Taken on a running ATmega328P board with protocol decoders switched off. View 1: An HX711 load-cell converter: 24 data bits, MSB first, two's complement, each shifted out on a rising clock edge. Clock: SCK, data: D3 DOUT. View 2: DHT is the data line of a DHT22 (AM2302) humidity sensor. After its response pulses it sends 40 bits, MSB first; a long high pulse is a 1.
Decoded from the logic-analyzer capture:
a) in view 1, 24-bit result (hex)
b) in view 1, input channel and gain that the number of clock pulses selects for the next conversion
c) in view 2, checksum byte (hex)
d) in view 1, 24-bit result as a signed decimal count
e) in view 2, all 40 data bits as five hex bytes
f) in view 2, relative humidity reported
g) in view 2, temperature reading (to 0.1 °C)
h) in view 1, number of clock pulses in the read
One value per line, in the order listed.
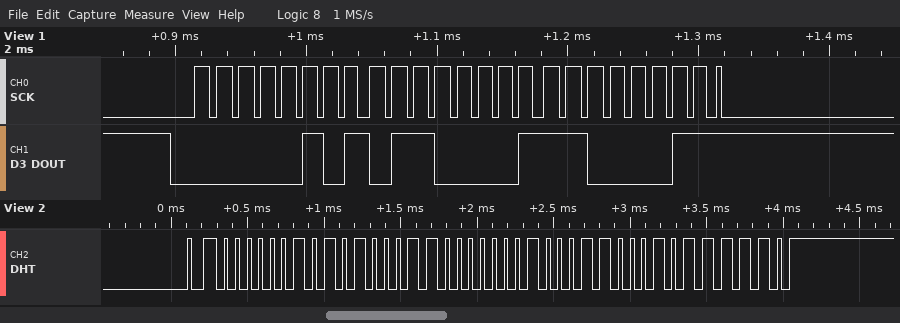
0x0561C3
channel A, gain 128
0xBE
352707
02 A3 01 18 BE
67.5 %
28.0 °C
25
